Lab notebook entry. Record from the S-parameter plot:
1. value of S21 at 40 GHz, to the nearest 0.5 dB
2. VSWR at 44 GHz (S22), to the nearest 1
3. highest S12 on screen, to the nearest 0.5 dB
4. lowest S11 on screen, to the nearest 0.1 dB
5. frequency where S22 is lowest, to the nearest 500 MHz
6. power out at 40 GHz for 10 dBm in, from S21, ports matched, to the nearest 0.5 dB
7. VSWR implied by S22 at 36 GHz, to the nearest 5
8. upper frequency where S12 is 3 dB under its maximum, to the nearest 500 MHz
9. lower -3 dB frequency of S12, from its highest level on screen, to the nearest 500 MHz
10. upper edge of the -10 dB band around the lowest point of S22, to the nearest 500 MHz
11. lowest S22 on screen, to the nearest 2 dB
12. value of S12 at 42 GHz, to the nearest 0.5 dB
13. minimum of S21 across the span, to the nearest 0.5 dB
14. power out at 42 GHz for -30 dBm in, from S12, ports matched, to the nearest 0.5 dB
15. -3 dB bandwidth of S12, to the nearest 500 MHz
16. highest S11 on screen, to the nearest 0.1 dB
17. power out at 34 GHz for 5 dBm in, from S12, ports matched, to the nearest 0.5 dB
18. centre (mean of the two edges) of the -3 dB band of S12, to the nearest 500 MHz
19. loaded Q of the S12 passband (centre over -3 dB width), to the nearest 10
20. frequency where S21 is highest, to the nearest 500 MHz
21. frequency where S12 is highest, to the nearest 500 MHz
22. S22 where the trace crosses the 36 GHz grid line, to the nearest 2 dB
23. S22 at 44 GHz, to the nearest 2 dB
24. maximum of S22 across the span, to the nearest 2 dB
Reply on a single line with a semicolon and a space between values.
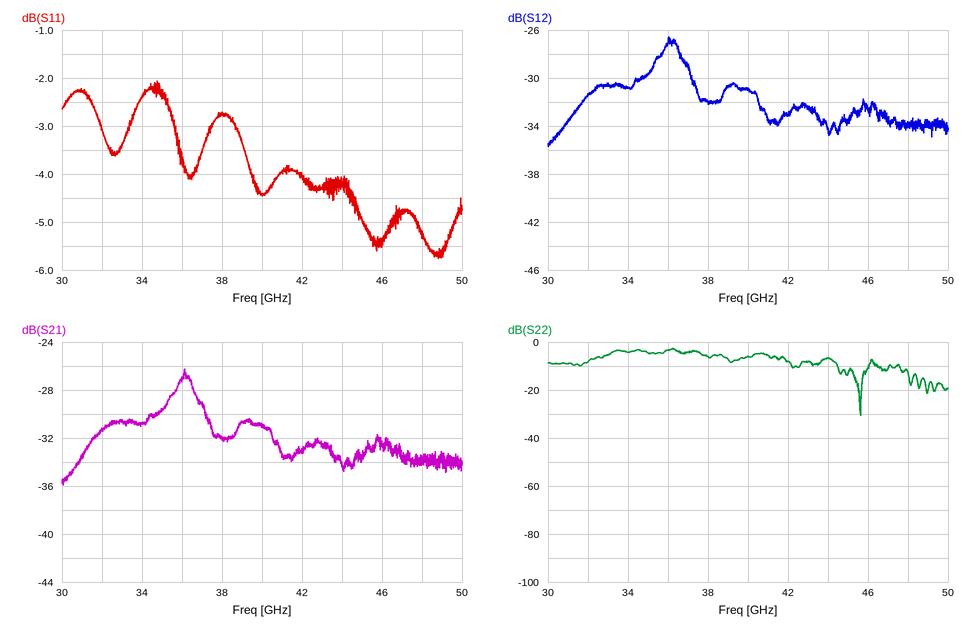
-31.0 dB; 3; -26.5 dB; -5.8 dB; 45.5 GHz; -21.0 dBm; 5; 37.0 GHz; 35.0 GHz; 46.0 GHz; -30 dB; -33.0 dB; -36.0 dB; -63.0 dBm; 2.0 GHz; -2.1 dB; -26.0 dBm; 36.0 GHz; 20; 36.0 GHz; 36.0 GHz; -4 dB; -6 dB; -2 dB
